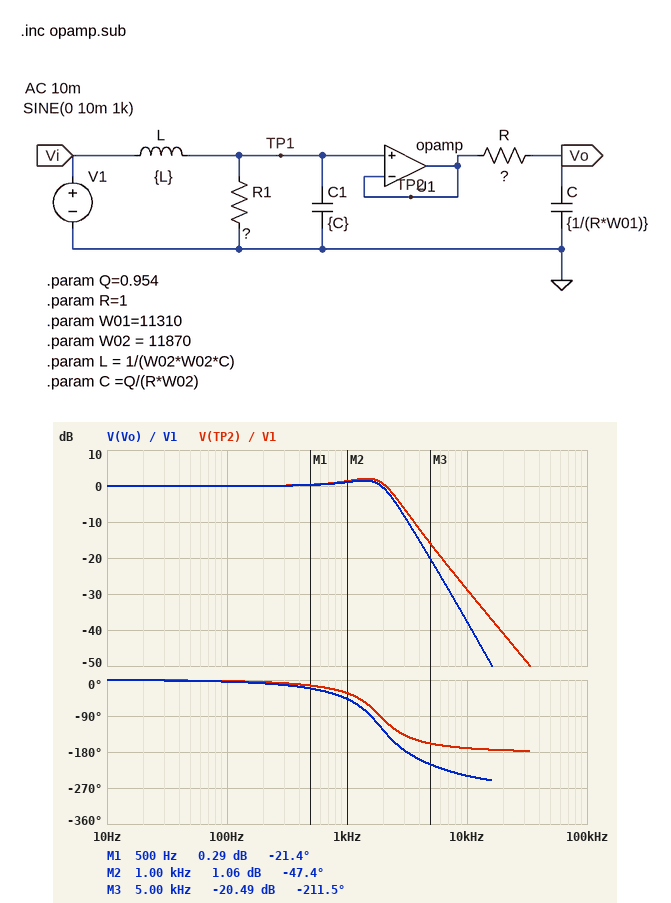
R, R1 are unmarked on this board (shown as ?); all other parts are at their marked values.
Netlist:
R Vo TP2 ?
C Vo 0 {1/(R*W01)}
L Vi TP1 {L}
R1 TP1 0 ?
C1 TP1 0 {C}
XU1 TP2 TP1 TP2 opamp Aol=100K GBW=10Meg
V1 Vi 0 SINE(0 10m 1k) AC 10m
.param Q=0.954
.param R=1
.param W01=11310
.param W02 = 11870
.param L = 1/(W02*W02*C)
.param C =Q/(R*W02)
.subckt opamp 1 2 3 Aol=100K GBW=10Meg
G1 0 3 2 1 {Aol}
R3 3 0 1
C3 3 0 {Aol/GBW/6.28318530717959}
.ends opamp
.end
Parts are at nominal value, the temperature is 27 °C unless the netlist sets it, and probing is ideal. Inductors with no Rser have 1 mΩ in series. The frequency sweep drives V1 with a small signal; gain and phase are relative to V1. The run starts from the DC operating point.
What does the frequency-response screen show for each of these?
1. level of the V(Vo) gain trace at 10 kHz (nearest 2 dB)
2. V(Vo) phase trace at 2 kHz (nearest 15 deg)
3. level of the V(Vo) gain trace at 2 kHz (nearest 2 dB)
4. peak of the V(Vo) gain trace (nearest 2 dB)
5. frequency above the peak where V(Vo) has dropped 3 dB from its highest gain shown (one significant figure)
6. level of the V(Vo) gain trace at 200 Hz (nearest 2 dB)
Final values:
-38 dB
-120 deg
0 dB
2 dB
2 kHz
0 dB
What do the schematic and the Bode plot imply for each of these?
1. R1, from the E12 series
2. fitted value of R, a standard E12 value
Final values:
1.2 Ω
0.47 Ω
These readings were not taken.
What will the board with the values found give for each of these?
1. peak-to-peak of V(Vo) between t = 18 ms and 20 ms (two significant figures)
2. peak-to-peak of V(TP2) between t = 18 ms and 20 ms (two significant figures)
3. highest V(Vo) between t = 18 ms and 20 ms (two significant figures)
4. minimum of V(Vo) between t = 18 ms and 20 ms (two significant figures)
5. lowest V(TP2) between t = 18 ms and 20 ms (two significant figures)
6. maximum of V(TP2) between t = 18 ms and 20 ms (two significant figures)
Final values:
23 mV
23 mV
11 mV
-11 mV
-12 mV
12 mV
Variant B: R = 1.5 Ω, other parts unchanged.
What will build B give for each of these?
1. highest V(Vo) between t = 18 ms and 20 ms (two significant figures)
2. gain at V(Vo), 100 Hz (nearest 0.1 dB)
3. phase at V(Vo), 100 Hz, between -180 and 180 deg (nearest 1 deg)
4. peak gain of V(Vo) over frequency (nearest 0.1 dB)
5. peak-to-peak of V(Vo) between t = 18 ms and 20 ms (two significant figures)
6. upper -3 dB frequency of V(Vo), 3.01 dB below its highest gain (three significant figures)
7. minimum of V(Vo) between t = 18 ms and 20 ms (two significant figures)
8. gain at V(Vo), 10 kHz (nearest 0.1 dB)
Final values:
9.0 mV
0 dB
-7 deg
0 dB
18 mV
1.71 kHz
-9.0 mV
-47.2 dB
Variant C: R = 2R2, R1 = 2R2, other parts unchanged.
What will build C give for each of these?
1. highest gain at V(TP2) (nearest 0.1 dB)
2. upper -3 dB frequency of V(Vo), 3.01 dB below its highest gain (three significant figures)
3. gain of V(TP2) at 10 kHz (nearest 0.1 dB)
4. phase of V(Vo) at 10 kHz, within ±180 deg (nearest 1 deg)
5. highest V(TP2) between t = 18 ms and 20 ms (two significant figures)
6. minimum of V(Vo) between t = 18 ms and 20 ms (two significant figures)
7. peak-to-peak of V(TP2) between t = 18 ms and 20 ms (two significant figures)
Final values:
6.7 dB
2.02 kHz
-28.7 dB
100 deg
13 mV
-8.3 mV
26 mV
